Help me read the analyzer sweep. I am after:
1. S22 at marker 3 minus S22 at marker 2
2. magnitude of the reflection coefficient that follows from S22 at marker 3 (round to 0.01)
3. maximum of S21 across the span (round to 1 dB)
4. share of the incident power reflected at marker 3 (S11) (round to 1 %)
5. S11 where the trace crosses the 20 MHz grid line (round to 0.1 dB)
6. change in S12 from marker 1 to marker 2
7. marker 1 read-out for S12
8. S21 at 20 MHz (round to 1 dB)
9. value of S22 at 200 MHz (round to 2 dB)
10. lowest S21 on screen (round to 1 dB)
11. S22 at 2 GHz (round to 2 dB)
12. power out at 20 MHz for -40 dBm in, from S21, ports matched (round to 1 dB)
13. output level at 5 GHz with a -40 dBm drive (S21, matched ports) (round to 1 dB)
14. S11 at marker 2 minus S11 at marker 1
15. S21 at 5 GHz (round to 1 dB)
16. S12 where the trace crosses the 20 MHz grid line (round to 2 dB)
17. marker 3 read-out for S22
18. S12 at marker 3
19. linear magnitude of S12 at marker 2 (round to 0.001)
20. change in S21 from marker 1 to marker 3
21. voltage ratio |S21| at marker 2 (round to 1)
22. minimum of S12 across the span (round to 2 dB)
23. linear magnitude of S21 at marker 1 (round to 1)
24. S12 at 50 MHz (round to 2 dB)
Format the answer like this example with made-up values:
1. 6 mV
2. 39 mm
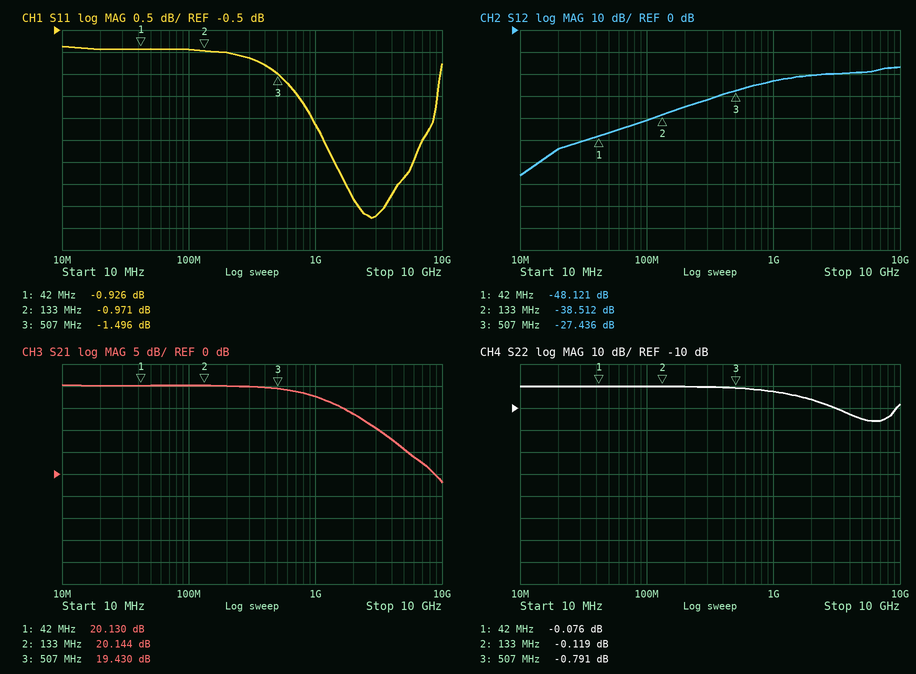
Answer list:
1. -0.672 dB
2. 0.91
3. 20 dB
4. 71 %
5. -0.9 dB
6. 9.609 dB
7. -48.121 dB
8. 20 dB
9. 0 dB
10. -2 dB
11. -6 dB
12. -20 dBm
13. -34 dBm
14. -0.045 dB
15. 6 dB
16. -54 dB
17. -0.791 dB
18. -27.436 dB
19. 0.012
20. -0.700 dB
21. 10
22. -66 dB
23. 10
24. -46 dB
